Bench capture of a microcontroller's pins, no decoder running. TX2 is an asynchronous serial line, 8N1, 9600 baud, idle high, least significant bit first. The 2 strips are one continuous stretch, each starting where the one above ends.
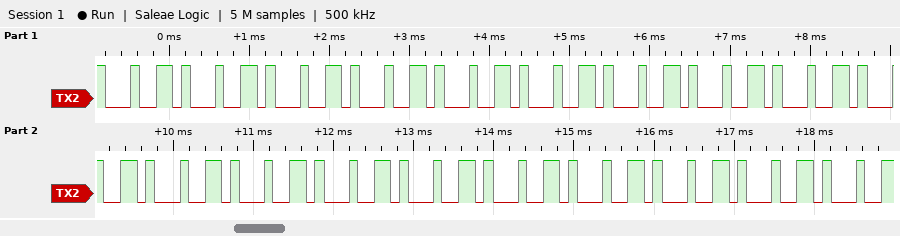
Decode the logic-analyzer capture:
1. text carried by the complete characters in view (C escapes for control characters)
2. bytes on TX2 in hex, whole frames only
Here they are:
"dddddddddddddddddd"
0x64 0x64 0x64 0x64 0x64 0x64 0x64 0x64 0x64 0x64 0x64 0x64 0x64 0x64 0x64 0x64 0x64 0x64
